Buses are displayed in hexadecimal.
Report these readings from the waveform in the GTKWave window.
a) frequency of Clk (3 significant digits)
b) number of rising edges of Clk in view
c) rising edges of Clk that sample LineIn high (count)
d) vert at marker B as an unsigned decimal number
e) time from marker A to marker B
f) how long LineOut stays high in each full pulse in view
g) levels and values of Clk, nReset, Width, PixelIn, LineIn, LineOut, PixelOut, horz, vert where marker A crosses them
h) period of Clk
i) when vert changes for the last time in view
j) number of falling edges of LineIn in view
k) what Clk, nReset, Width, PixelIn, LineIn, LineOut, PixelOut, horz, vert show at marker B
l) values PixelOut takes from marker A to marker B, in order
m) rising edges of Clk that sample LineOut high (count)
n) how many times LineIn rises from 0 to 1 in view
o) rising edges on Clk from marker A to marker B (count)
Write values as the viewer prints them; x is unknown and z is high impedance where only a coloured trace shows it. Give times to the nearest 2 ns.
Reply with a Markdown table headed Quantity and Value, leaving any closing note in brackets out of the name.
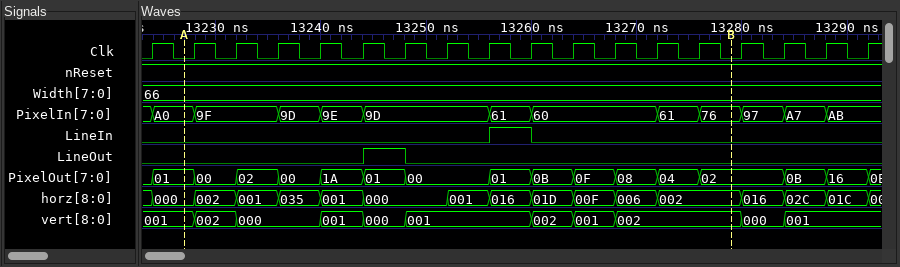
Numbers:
| Quantity | Value |
|---|---|
| frequency of Clk | 250 MHz |
| number of rising edges of Clk in view | 18 |
| rising edges of Clk that sample LineIn high | 1 |
| vert at marker B as an unsigned decimal number | 2 |
| time from marker A to marker B | 52 ns |
| how long LineOut stays high in each full pulse in view | 4 ns |
| levels and values of Clk, nReset, Width, PixelIn, LineIn, LineOut, PixelOut, horz, vert where marker A crosses them | Clk=0, nReset=1, Width=66, PixelIn=A0, LineIn=0, LineOut=0, PixelOut=01, horz=000, vert=001 |
| period of Clk | 4 ns |
| when vert changes for the last time in view | 13284 ns |
| number of falling edges of LineIn in view | 1 |
| what Clk, nReset, Width, PixelIn, LineIn, LineOut, PixelOut, horz, vert show at marker B | Clk=0, nReset=1, Width=66, PixelIn=76, LineIn=0, LineOut=0, PixelOut=02, horz=002, vert=002 |
| values PixelOut takes from marker A to marker B, in order | 01, 00, 02, 00, 1A, 01, 00, 01, 0B, 0F, 08, 04, 02 |
| rising edges of Clk that sample LineOut high | 1 |
| how many times LineIn rises from 0 to 1 in view | 1 |
| rising edges on Clk from marker A to marker B | 13 |
